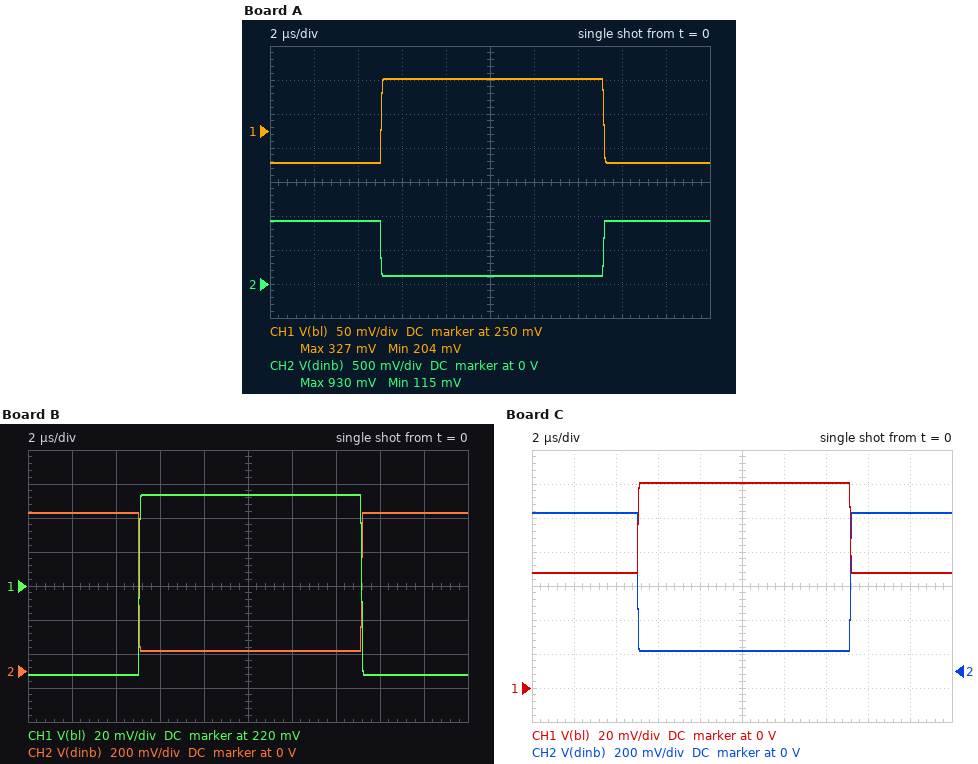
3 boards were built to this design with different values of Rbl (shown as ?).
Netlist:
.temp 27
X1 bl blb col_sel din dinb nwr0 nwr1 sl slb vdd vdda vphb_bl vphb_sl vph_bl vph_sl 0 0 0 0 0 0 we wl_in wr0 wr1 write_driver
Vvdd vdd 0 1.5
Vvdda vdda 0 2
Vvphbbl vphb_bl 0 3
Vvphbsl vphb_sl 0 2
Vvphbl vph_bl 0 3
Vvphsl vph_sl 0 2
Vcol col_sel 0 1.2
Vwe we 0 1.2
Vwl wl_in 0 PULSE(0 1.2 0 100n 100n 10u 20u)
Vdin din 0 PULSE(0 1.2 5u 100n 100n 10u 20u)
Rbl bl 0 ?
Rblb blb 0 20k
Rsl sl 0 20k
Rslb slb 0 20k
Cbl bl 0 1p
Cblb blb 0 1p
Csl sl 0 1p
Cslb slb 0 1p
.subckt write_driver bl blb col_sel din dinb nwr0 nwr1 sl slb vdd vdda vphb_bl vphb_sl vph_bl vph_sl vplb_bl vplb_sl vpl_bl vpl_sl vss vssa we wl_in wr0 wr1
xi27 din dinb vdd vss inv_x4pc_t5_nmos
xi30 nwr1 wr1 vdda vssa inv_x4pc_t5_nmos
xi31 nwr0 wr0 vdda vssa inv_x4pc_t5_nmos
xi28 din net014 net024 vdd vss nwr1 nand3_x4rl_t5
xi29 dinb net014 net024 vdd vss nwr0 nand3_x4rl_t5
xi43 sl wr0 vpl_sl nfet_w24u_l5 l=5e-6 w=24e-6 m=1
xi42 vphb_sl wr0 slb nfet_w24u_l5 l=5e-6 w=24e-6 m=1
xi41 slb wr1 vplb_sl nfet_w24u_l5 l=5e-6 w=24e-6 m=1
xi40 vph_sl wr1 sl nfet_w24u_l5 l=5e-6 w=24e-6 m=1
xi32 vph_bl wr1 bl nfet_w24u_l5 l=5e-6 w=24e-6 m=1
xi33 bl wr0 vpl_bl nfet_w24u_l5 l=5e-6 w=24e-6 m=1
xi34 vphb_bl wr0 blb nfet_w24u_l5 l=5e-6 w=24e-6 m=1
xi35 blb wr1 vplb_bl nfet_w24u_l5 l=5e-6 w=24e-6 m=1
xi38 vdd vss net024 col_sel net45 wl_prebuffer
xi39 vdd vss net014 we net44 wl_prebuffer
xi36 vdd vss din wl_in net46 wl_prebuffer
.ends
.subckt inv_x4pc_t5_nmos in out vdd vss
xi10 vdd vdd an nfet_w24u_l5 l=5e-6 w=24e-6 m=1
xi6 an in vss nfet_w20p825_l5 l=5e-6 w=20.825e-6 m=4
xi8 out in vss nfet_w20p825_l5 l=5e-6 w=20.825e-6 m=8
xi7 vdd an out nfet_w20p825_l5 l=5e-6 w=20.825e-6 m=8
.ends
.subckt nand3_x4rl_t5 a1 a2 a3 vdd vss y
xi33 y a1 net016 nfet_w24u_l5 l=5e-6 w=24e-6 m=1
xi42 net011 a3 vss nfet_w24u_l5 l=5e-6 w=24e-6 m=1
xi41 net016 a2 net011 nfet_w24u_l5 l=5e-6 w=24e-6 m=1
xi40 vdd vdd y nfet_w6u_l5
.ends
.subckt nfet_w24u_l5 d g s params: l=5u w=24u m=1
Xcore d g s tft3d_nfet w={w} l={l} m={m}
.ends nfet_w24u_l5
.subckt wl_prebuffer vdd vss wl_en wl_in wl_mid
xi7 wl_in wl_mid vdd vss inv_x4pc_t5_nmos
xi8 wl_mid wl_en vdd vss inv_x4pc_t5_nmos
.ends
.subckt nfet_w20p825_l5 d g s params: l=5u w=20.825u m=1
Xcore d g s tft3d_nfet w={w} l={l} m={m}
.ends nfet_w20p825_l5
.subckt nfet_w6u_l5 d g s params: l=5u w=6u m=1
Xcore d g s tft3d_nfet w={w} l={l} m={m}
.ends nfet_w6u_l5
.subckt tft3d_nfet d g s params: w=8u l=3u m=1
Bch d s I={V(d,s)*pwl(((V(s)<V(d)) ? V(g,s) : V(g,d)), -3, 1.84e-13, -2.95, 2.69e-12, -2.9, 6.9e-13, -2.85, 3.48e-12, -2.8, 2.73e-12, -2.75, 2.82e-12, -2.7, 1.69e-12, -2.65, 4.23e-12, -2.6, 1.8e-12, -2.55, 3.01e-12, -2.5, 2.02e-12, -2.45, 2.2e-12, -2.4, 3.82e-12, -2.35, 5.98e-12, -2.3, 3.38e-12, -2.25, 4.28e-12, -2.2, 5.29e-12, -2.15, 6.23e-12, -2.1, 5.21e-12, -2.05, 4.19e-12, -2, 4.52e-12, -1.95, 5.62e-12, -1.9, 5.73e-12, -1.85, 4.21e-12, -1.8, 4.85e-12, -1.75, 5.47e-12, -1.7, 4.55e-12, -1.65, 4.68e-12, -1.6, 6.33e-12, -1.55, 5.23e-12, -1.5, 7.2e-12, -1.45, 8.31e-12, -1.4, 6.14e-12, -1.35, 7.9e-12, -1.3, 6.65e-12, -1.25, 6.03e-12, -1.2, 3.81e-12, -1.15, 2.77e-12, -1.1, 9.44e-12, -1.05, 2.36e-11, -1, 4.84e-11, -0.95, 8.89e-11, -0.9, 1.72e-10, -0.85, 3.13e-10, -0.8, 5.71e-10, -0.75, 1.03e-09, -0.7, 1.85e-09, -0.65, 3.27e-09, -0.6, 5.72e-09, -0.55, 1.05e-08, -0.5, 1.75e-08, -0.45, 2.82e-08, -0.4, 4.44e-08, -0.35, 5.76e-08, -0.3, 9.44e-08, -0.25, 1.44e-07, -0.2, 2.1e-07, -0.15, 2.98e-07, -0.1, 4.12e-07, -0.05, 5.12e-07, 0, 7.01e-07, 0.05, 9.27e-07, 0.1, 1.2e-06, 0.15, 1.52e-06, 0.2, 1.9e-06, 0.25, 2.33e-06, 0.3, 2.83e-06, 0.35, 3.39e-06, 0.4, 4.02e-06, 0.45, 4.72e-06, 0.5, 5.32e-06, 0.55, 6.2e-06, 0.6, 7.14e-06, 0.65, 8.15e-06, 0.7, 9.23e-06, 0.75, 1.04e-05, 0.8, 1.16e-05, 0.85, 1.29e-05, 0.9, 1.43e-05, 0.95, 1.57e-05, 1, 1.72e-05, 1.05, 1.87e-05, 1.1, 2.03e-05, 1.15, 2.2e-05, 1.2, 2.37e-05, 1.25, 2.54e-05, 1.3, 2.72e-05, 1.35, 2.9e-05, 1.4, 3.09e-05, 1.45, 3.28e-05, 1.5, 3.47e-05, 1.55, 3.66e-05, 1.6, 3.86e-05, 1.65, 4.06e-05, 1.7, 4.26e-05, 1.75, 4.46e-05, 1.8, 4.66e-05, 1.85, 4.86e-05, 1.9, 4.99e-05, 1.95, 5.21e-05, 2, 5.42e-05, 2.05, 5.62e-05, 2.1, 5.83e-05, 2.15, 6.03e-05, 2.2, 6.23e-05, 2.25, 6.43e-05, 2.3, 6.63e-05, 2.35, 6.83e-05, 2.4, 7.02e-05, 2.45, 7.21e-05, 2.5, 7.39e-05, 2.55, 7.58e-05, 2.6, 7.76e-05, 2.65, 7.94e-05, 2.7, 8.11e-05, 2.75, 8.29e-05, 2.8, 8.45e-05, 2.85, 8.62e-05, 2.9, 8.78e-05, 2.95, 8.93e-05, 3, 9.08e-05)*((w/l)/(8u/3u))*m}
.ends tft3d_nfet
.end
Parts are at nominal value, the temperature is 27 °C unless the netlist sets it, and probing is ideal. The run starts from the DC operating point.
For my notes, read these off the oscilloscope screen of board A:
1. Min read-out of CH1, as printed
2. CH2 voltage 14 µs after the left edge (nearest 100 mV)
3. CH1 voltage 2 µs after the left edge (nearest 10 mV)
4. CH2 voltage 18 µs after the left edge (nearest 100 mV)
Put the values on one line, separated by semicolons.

204 mV; 100 mV; 200 mV; 900 mV
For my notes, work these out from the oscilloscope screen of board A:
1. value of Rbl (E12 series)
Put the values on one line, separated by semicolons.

56 kΩ
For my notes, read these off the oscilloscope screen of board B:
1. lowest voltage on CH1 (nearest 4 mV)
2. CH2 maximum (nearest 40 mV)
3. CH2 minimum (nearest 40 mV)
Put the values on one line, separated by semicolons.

168 mV; 920 mV; 120 mV
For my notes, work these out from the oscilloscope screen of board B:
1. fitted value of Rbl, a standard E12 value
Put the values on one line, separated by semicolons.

33 kΩ
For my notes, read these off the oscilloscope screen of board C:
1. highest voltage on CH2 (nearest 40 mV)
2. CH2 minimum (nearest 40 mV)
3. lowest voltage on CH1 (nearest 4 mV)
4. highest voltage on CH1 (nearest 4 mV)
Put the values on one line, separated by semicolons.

920 mV; 120 mV; 68 mV; 120 mV
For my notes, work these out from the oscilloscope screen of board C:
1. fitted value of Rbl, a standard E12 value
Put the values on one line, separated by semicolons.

6.8 kΩ
